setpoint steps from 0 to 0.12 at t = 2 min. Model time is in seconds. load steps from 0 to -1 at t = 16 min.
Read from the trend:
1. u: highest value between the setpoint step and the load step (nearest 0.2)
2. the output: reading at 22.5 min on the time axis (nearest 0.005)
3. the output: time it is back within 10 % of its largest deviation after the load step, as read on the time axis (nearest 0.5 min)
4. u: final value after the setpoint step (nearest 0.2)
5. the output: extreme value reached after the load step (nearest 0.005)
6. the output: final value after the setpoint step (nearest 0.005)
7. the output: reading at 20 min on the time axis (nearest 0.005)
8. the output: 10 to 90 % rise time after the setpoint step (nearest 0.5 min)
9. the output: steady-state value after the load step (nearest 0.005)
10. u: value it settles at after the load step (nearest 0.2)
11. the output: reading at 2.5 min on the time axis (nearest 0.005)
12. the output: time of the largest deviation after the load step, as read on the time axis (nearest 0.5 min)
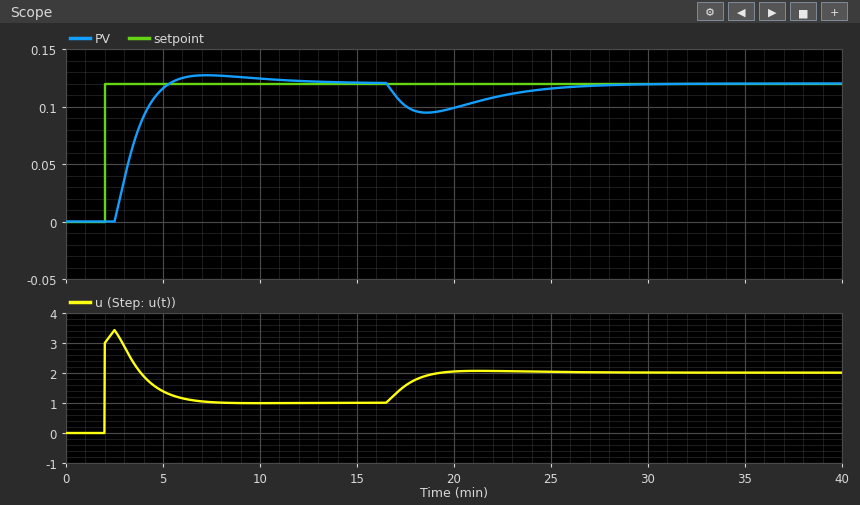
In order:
3.4
0.110
26.5 min
1.0
0.095
0.120
0.100
2.0 min
0.120
2.0
0.000
18.5 min
